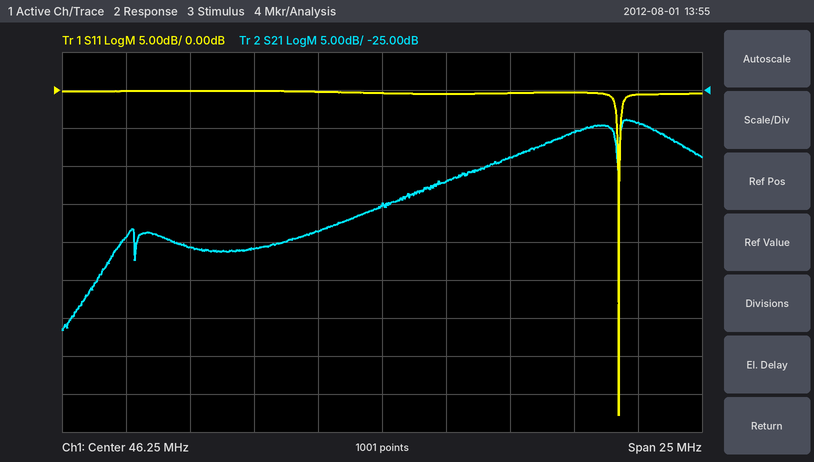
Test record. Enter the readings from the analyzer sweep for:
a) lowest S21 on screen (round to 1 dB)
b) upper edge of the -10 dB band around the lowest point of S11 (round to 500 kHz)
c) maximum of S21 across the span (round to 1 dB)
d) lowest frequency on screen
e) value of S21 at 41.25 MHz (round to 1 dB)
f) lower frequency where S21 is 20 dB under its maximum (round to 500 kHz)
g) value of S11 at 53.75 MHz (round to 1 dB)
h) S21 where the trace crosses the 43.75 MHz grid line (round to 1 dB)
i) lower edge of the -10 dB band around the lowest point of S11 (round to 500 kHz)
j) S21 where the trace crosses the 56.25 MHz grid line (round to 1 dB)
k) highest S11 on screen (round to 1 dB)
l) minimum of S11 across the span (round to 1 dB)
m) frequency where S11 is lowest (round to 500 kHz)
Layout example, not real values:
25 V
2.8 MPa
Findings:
-57 dB
55.5 MHz
-29 dB
33.75 MHz
-46 dB
35.5 MHz
0 dB
-44 dB
55.5 MHz
-29 dB
0 dB
-43 dB
55.5 MHz
